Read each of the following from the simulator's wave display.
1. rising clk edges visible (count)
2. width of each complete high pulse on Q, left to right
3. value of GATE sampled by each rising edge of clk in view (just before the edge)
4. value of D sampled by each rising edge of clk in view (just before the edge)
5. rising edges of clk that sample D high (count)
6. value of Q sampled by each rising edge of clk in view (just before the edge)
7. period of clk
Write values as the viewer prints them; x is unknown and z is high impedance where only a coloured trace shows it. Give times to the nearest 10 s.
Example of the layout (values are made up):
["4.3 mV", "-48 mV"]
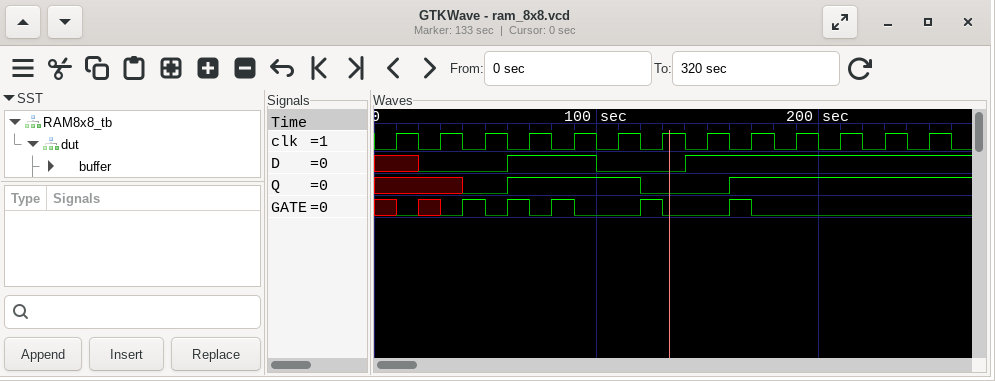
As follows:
["13", "60 s", "x x 1 1 1 0 1 0 1 0 0 0 0", "x 0 0 1 1 0 0 1 1 1 1 1 1", "8", "x x 0 1 1 1 0 0 1 1 1 1 1", "20 s"]
